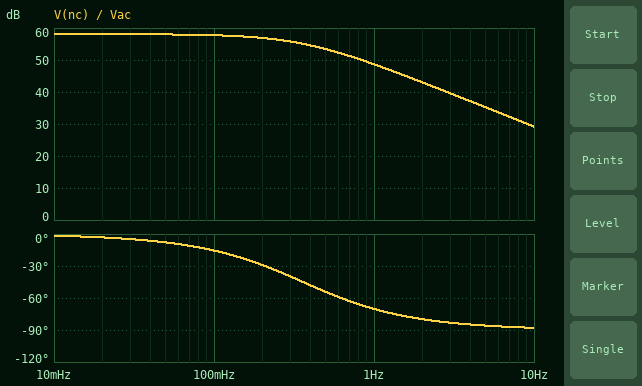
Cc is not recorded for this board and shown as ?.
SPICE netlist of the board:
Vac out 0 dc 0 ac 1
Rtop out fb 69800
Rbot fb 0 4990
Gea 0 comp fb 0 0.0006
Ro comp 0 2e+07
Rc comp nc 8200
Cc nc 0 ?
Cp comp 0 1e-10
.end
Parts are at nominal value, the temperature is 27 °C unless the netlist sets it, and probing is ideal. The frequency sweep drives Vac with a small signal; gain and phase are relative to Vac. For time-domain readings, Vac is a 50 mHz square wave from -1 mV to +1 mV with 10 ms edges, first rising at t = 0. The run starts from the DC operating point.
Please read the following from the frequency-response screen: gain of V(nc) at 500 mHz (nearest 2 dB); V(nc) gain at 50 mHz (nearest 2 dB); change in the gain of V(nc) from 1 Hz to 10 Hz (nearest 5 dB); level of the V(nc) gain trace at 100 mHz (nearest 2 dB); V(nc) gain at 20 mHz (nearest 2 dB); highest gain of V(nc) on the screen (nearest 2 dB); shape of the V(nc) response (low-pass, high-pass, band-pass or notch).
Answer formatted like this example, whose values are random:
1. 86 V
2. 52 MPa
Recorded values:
1. 54 dB
2. 58 dB
3. -20 dB
4. 58 dB
5. 58 dB
6. 58 dB
7. low-pass
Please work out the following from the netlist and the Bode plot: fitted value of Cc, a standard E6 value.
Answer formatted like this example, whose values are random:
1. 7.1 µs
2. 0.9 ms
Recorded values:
1. 22 nF
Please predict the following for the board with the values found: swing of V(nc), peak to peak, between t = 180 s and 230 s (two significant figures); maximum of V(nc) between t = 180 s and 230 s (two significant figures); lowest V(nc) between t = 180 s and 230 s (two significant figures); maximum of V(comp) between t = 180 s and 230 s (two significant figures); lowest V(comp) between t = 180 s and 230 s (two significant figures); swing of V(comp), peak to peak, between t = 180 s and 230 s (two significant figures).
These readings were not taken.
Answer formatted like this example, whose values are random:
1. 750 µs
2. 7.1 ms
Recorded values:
1. 1.6 V
2. 800 mV
3. -800 mV
4. 800 mV
5. -800 mV
6. 1.6 V
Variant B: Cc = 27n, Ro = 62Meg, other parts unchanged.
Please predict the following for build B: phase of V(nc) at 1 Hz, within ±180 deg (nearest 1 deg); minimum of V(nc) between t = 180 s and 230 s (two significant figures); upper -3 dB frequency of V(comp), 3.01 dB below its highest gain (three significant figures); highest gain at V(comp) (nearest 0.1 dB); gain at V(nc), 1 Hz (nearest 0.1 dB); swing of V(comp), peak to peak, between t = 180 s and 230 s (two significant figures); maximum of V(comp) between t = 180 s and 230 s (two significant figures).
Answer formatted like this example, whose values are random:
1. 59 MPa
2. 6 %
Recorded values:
1. -85 deg
2. -2.5 V
3. 94.7 mHz
4. 67.9 dB
5. 47.4 dB
6. 4.9 V
7. 2.5 V
